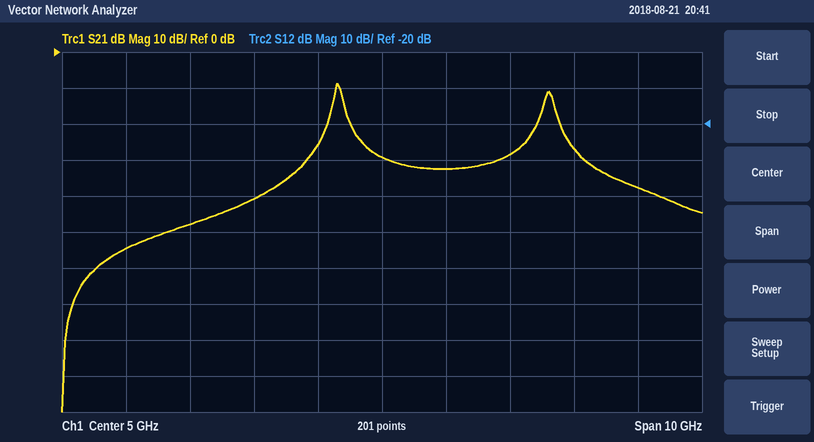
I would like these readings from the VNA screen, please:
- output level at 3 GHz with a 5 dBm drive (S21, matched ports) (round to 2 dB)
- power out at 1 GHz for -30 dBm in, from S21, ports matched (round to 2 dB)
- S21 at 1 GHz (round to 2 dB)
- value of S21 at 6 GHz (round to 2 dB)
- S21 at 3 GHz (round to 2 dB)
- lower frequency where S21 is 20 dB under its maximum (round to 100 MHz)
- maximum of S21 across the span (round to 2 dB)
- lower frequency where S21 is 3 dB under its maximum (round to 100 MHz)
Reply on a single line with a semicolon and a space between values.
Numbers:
-36 dBm; -84 dBm; -54 dB; -32 dB; -40 dB; 3.9 GHz; -8 dB; 4.3 GHz
